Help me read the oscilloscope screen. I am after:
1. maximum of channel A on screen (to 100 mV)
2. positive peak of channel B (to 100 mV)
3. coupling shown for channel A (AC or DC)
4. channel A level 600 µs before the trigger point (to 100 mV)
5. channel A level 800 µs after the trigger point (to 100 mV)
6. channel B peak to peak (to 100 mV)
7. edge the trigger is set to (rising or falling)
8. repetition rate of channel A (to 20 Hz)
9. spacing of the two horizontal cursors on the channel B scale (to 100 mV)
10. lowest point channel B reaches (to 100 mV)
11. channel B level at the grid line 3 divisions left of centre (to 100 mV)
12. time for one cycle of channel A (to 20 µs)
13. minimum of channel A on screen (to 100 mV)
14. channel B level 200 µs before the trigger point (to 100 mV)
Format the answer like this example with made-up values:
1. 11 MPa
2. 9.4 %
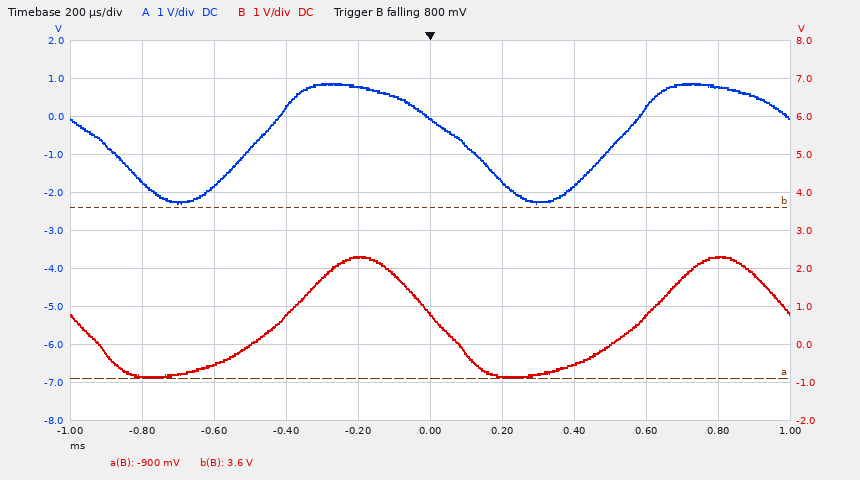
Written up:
1. 900 mV
2. 2.3 V
3. DC
4. -1.8 V
5. 800 mV
6. 3.2 V
7. falling
8. 1.00 kHz
9. 4.5 V
10. -900 mV
11. -500 mV
12. 1.00 ms
13. -2.3 V
14. 2.3 V
